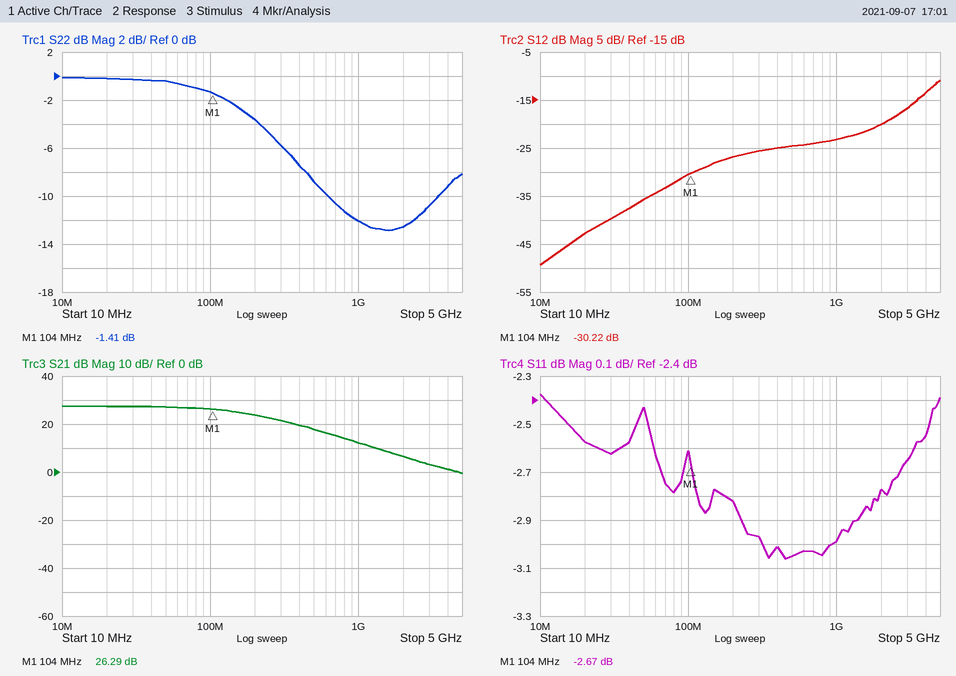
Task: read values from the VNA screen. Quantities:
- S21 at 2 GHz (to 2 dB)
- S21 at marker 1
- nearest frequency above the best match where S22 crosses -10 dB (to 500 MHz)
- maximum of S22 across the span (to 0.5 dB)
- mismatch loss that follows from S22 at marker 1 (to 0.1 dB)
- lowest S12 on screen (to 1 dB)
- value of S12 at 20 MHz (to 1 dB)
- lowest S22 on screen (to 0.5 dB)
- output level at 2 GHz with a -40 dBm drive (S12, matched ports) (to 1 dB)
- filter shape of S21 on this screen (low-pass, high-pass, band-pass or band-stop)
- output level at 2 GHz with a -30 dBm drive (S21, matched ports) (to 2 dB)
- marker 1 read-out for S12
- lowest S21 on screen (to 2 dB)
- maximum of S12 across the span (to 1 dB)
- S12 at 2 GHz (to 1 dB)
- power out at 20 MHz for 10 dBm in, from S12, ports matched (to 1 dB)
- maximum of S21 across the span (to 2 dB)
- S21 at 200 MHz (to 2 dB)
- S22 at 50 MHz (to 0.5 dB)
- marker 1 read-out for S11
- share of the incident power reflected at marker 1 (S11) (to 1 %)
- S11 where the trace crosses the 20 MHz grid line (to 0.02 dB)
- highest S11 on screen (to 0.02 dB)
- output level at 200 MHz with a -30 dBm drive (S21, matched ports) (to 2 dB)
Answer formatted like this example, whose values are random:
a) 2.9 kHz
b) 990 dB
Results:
a) 6 dB
b) 26.29 dB
c) 3.5 GHz
d) 0.0 dB
e) 5.6 dB
f) -49 dB
g) -43 dB
h) -13.0 dB
i) -60 dBm
j) low-pass
k) -24 dBm
l) -30.22 dB
m) 0 dB
n) -11 dB
o) -20 dB
p) -33 dBm
q) 28 dB
r) 24 dB
s) -0.5 dB
t) -2.67 dB
u) 54 %
v) -2.58 dB
w) -2.38 dB
x) -6 dBm
